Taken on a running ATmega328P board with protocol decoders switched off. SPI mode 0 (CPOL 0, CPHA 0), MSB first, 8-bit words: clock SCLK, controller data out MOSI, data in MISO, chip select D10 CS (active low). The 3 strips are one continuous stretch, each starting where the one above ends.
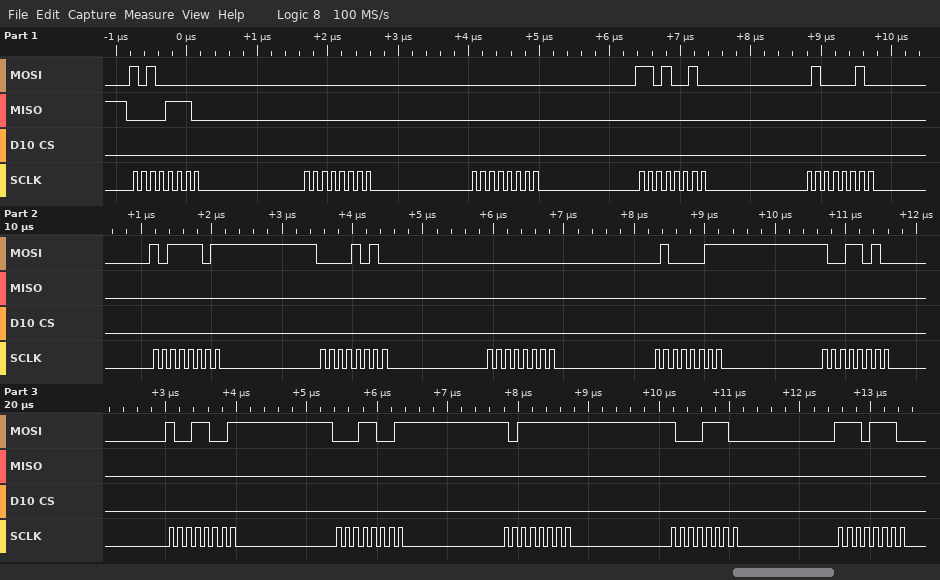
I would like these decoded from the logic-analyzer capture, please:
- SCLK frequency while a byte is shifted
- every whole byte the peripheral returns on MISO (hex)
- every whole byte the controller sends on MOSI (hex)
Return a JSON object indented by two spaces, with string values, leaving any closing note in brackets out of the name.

{
  "SCLK frequency while a byte is shifted": "8 MHz",
  "every whole byte the peripheral returns on MISO": "0x0E 0x00 0x00 0x00 0x00 0x00 0x00 0x00 0x00 0x00 0x00 0x00 0x00 0x00 0x00",
  "every whole byte the controller sends on MOSI": "0xA0 0x00 0x00 0xD2 0x42 0xBD 0x0A 0x00 0x43 0x9A 0x99 0x19 0xBF 0x8E 0xEE"
}
